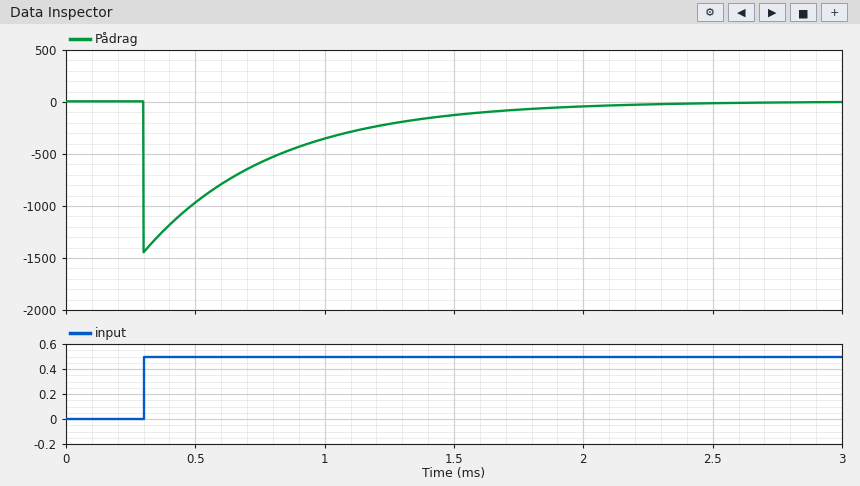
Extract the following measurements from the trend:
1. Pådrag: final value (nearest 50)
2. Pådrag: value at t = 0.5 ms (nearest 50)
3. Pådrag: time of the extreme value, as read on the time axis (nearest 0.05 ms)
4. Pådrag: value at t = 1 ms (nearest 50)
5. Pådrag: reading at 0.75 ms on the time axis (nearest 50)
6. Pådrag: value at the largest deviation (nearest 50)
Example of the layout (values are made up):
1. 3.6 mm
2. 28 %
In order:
1. 0
2. -950
3. 0.30 ms
4. -350
5. -600
6. -1450
